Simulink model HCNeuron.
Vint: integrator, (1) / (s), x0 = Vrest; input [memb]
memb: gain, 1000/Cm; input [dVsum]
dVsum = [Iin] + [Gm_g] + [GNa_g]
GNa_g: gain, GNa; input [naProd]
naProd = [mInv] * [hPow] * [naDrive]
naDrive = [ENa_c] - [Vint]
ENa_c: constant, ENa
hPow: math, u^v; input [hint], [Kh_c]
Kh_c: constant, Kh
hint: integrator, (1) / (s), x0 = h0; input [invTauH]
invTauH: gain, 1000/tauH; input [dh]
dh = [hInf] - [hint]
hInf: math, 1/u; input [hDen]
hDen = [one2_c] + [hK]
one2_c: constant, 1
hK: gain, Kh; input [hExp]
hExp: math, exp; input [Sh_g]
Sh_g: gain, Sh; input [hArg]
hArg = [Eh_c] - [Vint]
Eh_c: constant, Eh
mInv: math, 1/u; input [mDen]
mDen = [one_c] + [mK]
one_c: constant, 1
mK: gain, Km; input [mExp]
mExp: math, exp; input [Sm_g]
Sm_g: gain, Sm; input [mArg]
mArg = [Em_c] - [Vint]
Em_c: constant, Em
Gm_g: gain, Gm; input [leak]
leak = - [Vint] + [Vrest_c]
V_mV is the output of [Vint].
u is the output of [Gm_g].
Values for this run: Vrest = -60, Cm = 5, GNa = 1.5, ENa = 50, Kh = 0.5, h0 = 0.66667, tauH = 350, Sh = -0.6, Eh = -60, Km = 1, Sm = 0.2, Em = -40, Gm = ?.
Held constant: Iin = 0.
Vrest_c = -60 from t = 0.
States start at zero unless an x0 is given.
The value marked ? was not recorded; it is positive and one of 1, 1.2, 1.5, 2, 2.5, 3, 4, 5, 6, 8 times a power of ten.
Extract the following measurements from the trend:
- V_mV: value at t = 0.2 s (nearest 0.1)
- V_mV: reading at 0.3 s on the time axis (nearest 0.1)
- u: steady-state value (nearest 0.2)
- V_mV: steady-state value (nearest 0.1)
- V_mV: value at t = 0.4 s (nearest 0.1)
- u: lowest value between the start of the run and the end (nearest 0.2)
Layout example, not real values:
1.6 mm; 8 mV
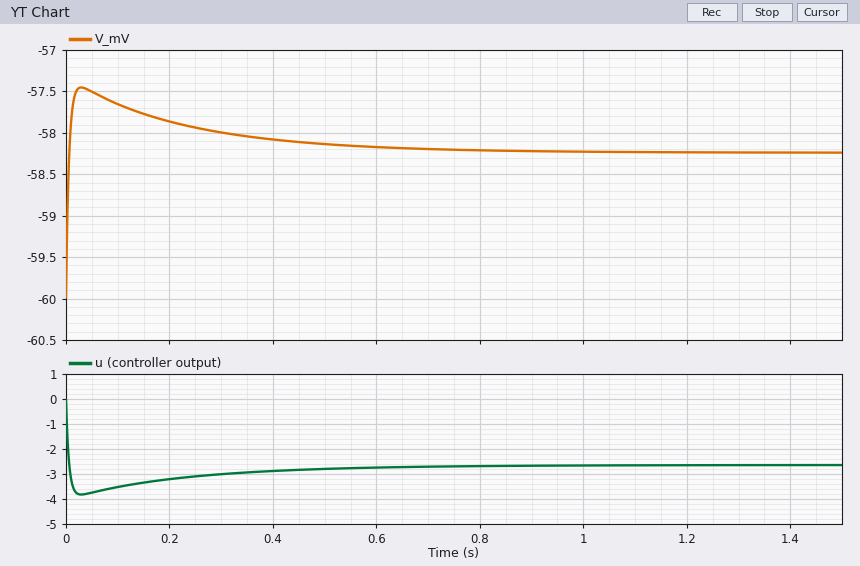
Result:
-57.9; -58.0; -2.6; -58.2; -58.1; -3.8
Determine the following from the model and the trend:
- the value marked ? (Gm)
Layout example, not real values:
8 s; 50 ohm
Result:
1.5
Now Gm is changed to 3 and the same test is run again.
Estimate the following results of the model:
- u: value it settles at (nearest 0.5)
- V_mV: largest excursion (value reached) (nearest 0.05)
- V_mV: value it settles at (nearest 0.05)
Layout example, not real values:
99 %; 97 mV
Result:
-2.5; -59.05; -59.15
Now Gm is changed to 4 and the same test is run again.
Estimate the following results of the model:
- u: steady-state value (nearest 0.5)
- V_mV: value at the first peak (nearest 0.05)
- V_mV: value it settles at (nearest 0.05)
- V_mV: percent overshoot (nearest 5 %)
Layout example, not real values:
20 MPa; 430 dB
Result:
-2.5; -59.30; -59.35; 10 %
